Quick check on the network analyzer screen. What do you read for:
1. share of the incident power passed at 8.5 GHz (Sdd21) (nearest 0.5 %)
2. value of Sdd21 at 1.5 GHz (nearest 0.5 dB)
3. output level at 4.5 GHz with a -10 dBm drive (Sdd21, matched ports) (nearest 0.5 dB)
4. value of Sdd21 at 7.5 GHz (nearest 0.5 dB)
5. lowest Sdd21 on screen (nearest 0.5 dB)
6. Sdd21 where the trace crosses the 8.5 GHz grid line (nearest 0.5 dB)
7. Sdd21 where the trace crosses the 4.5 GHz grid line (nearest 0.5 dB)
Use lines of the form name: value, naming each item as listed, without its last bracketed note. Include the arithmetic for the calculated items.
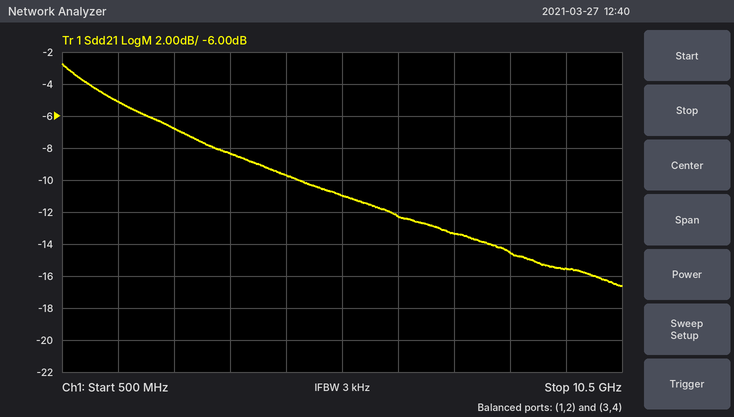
share of the incident power passed at 8.5 GHz (Sdd21): 10^(-14.5/10) ≈ 3.5 %
value of Sdd21 at 1.5 GHz: -5.0 dB
output level at 4.5 GHz with a -10 dBm drive (Sdd21, matched ports): -10 dBm + (-9.5 dB) = -19.5 dBm
value of Sdd21 at 7.5 GHz: -13.5 dB
lowest Sdd21 on screen: -16.5 dB
Sdd21 where the trace crosses the 8.5 GHz grid line: -14.5 dB
Sdd21 where the trace crosses the 4.5 GHz grid line: -9.5 dB
